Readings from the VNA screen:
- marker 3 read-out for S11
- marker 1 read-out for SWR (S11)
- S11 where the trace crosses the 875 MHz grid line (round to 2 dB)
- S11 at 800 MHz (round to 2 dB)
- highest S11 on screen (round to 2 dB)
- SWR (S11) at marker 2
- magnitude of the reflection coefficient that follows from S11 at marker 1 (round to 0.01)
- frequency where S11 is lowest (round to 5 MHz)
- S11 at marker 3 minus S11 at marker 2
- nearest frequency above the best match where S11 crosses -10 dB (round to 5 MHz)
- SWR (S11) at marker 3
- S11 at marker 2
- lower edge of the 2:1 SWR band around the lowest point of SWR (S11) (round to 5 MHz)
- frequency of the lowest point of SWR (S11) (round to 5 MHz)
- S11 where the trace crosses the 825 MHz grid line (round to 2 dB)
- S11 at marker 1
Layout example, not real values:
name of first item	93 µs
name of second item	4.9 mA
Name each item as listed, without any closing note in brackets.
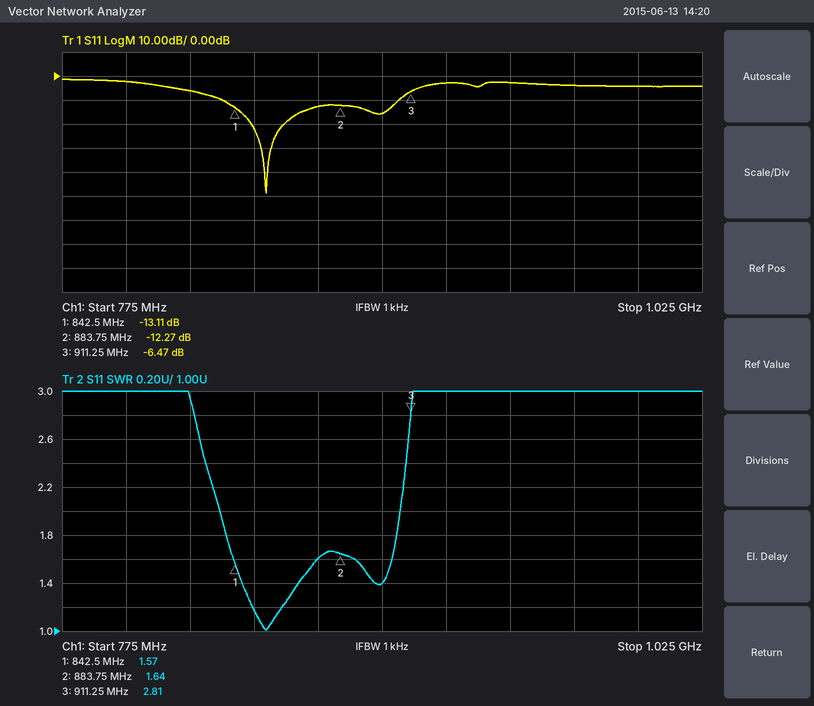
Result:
marker 3 read-out for S11	-6.47 dB
marker 1 read-out for SWR	1.57
S11 where the trace crosses the 875 MHz grid line	-12 dB
S11 at 800 MHz	-2 dB
highest S11 on screen	-2 dB
SWR (S11) at marker 2	1.64
magnitude of the reflection coefficient that follows from S11 at marker 1	0.22
frequency where S11 is lowest	855 MHz
S11 at marker 3 minus S11 at marker 2	5.80 dB
nearest frequency above the best match where S11 crosses -10 dB	905 MHz
SWR (S11) at marker 3	2.81
S11 at marker 2	-12.27 dB
lower edge of the 2:1 SWR band around the lowest point of SWR (S11)	835 MHz
frequency of the lowest point of SWR (S11)	855 MHz
S11 where the trace crosses the 825 MHz grid line	-6 dB
S11 at marker 1	-13.11 dB
